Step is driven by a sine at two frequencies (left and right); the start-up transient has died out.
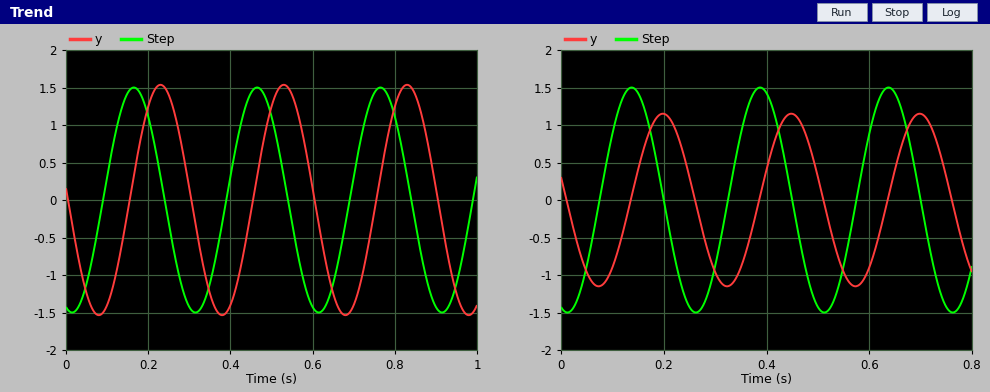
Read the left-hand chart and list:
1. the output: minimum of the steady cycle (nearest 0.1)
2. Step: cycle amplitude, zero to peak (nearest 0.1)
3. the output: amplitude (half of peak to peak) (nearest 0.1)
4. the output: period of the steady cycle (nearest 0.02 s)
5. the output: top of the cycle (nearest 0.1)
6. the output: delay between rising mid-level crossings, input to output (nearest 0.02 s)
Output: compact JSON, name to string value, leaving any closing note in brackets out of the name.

{"the output: minimum of the steady cycle": "-1.5", "Step: cycle amplitude, zero to peak": "1.5", "the output: amplitude (half of peak to peak)": "1.5", "the output: period of the steady cycle": "0.30 s", "the output: top of the cycle": "1.5", "the output: delay between rising mid-level crossings, input to output": "0.06 s"}
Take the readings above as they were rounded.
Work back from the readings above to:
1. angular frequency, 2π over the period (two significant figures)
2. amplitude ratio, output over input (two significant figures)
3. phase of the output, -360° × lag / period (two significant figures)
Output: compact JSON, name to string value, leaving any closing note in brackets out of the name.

{"angular frequency, 2π over the period": "21 rad/s", "amplitude ratio, output over input": "1.0", "phase of the output, -360° × lag / period": "-72°"}
